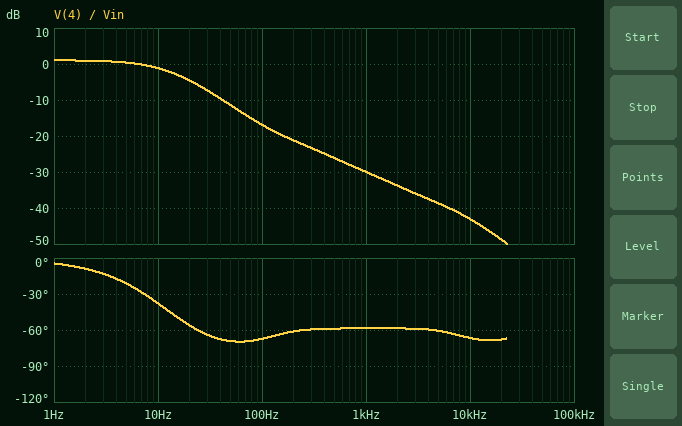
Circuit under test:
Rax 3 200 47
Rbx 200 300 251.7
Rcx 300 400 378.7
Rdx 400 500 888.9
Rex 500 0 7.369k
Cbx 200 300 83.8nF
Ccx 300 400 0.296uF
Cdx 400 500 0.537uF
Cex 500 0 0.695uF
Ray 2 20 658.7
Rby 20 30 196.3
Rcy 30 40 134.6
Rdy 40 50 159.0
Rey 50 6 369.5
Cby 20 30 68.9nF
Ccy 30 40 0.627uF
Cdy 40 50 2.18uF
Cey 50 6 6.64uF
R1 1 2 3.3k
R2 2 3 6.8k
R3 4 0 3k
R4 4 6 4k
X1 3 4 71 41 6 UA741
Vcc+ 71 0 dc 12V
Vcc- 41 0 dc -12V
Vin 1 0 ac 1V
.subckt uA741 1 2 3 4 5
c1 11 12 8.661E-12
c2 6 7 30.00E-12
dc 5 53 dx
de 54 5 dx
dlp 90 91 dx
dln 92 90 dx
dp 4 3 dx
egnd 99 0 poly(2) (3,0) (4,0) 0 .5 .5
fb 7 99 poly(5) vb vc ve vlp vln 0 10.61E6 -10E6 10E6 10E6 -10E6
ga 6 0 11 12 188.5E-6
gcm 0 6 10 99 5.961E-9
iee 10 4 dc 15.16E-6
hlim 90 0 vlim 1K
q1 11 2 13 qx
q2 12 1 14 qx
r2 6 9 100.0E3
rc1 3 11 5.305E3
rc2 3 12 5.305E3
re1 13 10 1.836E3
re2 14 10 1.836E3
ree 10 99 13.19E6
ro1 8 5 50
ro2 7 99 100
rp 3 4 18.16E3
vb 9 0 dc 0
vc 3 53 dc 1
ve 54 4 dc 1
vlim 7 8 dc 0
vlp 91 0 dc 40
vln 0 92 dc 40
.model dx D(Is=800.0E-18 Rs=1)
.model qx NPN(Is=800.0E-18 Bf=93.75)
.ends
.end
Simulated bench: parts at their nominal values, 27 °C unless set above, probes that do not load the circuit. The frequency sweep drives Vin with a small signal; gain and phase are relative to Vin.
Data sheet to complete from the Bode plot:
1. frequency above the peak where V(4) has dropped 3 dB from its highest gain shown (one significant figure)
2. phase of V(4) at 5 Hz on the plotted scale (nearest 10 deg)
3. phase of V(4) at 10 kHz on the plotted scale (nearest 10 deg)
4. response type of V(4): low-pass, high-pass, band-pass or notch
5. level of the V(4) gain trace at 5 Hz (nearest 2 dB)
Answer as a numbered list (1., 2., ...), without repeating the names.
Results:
1. 10 Hz
2. -20 deg
3. -70 deg
4. low-pass
5. 0 dB
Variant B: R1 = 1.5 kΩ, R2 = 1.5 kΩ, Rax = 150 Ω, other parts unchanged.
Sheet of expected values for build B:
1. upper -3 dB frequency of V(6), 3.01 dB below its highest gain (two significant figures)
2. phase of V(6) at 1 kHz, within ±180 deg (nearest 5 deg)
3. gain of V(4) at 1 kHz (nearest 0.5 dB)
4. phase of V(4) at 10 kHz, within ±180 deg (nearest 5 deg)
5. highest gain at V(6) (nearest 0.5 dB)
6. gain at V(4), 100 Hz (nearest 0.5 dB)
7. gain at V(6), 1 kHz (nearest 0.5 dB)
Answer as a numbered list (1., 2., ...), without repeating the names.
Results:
1. 20 Hz
2. -55 deg
3. -12.5 dB
4. -50 deg
5. 22.5 dB
6. 0.5 dB
7. -5.0 dB
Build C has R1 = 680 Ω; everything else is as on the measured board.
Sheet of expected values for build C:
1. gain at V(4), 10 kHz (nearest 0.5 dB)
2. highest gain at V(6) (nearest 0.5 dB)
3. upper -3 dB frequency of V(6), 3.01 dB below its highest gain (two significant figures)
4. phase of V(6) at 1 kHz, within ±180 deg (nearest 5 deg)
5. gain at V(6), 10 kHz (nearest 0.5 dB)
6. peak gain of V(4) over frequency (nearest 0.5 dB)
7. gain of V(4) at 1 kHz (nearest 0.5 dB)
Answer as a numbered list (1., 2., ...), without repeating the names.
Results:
1. -34.0 dB
2. 3.5 dB
3. 45 Hz
4. -50 deg
5. -26.5 dB
6. -4.0 dB
7. -22.0 dB
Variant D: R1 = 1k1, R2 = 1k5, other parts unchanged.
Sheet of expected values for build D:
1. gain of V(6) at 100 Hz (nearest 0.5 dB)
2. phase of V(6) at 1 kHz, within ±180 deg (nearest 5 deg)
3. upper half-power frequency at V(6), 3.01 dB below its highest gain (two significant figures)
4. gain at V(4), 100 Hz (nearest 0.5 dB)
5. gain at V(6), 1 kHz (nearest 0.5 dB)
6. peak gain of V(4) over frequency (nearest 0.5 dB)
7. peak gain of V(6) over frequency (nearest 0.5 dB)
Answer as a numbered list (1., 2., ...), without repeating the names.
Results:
1. 7.5 dB
2. -55 deg
3. 51 Hz
4. 0 dB
5. -4.5 dB
6. 7.0 dB
7. 14.5 dB
